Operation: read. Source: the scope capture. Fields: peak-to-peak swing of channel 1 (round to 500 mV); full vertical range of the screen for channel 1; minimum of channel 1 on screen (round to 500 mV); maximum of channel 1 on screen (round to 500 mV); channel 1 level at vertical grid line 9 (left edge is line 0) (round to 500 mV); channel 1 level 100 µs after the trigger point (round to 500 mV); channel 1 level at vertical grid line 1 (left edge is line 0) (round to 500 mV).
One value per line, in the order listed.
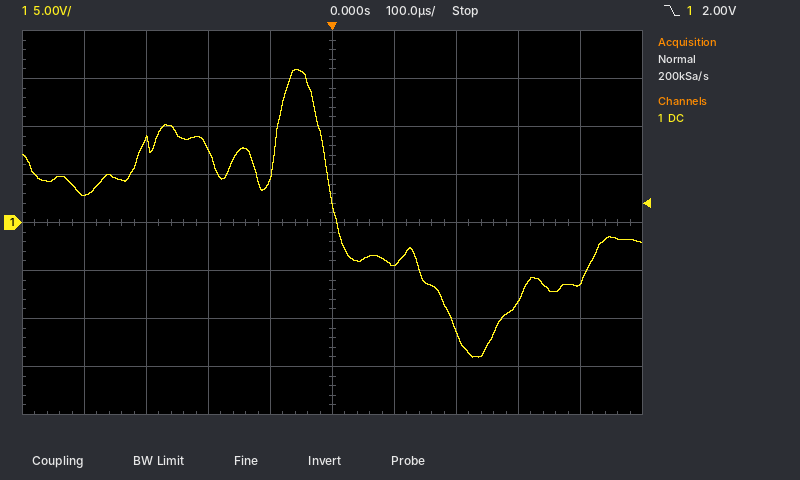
30.0 V
40 V
-14.0 V
16.0 V
-6.0 V
-4.5 V
3.0 V
